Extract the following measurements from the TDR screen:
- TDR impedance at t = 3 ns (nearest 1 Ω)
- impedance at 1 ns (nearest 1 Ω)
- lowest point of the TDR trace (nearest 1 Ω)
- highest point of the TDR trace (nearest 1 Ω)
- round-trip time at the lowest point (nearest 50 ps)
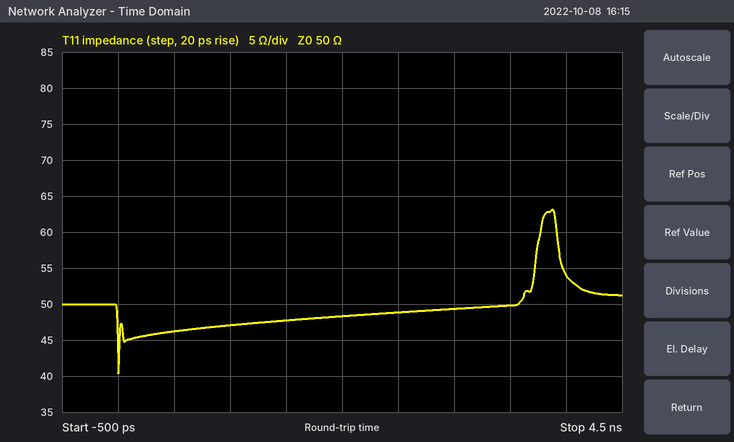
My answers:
49 Ω
47 Ω
40 Ω
63 Ω
0 ps
